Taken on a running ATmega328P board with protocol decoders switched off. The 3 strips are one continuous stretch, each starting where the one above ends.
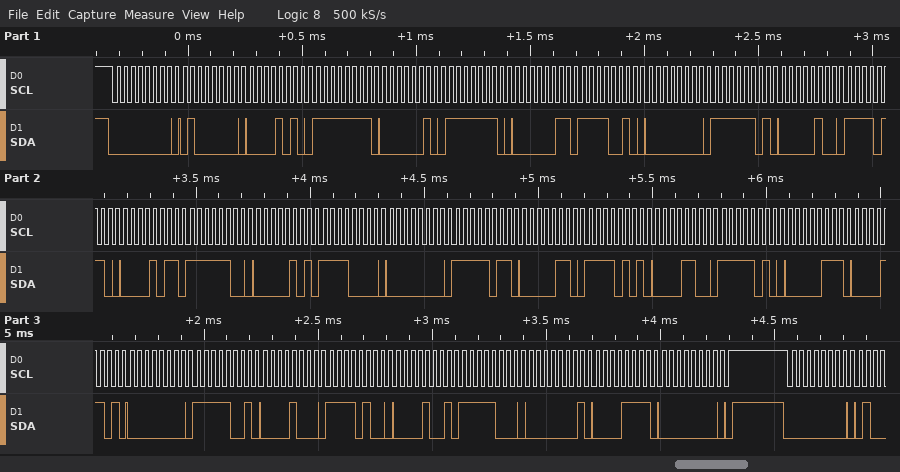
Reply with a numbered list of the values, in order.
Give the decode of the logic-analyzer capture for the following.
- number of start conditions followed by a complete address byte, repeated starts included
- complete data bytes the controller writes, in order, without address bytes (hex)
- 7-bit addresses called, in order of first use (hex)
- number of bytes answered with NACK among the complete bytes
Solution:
1. 2
2. 40 0A FF 02 FE 03 F2 00 FD 04 F6 0B FC 05 F0 00 FB 06 F5 0C FA 07 0D 00 F9 08 F4 09 F8 01 0F 00
3. 0x00
4. 0
